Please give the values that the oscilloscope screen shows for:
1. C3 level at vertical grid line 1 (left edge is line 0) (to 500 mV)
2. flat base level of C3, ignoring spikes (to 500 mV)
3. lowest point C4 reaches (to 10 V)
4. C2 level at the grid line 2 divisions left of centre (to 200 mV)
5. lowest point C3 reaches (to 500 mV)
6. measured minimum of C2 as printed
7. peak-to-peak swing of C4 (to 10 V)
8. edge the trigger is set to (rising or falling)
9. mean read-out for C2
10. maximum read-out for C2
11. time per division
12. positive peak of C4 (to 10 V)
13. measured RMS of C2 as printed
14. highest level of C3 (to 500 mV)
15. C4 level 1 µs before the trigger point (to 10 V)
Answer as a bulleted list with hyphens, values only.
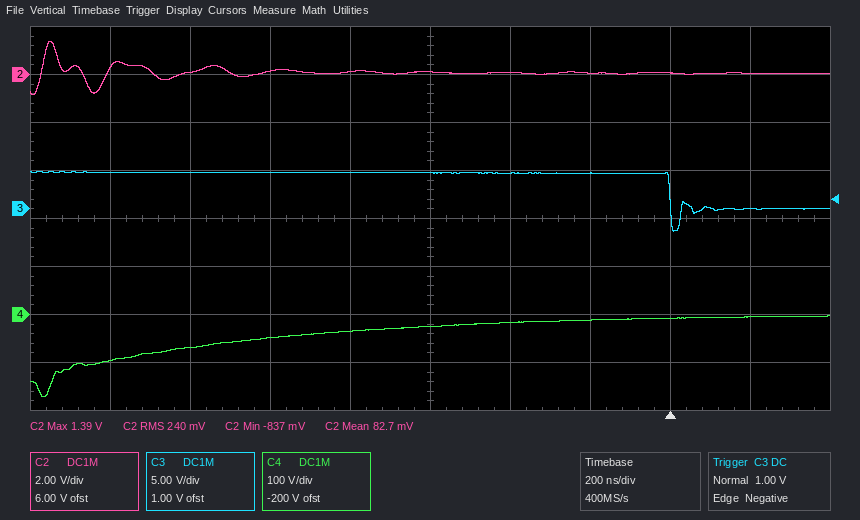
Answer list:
- 4.0 V
- 0.0 V
- -170 V
- 200 mV
- -2.5 V
- -837 mV
- 170 V
- falling
- 82.7 mV
- 1.39 V
- 200 ns
- 0 V
- 240 mV
- 4.0 V
- -50 V
